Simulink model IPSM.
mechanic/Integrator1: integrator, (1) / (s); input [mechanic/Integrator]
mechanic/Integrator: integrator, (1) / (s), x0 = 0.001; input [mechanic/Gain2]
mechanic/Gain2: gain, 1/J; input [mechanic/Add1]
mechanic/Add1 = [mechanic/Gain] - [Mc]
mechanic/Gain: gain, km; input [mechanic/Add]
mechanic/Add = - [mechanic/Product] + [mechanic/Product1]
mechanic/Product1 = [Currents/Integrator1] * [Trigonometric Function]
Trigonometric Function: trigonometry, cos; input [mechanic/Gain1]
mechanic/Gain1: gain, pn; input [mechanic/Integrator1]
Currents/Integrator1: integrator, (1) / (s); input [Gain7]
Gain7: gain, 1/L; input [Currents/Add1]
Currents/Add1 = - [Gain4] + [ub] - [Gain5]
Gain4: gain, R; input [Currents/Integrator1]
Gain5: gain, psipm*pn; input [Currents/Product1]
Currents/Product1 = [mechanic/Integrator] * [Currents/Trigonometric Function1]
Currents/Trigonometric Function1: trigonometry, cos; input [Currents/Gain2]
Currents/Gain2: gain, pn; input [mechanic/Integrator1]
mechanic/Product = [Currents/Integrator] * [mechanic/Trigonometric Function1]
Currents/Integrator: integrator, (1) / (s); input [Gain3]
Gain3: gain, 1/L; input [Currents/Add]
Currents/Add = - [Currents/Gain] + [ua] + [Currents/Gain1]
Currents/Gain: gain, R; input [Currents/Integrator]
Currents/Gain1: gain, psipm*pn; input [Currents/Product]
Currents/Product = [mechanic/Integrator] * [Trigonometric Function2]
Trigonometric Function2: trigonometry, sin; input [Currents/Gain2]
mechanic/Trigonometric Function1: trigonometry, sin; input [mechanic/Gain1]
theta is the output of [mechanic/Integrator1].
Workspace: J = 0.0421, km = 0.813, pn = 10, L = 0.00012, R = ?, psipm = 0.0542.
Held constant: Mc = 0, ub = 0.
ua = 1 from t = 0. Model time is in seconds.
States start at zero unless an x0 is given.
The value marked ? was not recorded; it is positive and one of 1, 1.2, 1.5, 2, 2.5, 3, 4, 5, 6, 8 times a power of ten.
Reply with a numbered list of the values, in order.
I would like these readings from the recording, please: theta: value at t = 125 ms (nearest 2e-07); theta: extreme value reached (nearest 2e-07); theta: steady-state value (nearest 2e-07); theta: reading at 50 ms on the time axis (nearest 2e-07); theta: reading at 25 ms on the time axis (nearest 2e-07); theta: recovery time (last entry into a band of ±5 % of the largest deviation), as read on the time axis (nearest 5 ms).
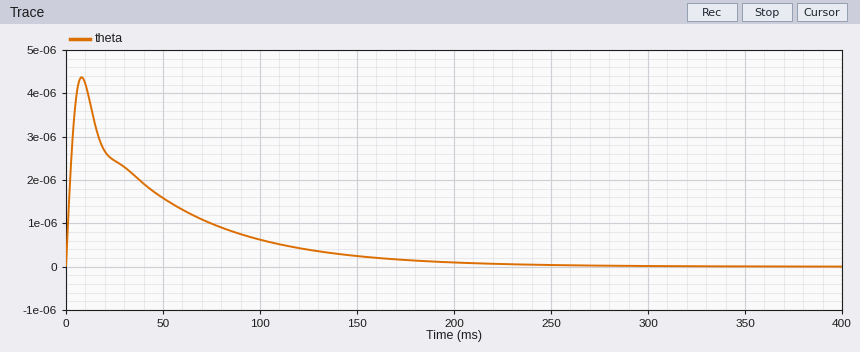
1. 0.0000004
2. 0.0000044
3. 0.0000000
4. 0.0000016
5. 0.0000024
6. 155 ms
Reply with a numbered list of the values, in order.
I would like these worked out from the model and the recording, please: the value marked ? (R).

1. 0.04
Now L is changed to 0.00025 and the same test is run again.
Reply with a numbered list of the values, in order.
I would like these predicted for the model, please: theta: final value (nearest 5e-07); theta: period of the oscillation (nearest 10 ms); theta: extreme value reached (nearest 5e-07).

1. 0.0000000
2. 30 ms
3. 0.0000055
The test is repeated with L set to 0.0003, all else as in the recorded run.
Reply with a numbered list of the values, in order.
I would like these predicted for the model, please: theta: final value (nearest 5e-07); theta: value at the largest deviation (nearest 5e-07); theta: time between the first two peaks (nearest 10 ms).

1. 0.0000000
2. 0.0000060
3. 30 ms
